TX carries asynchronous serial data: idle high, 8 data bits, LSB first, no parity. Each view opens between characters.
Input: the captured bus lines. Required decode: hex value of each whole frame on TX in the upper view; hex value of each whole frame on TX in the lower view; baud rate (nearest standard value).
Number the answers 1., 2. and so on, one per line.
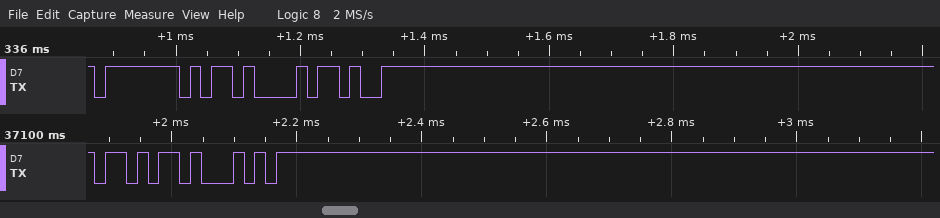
1. 7F, 0B, CB
2. 6B, D4
3. 57600 baud
